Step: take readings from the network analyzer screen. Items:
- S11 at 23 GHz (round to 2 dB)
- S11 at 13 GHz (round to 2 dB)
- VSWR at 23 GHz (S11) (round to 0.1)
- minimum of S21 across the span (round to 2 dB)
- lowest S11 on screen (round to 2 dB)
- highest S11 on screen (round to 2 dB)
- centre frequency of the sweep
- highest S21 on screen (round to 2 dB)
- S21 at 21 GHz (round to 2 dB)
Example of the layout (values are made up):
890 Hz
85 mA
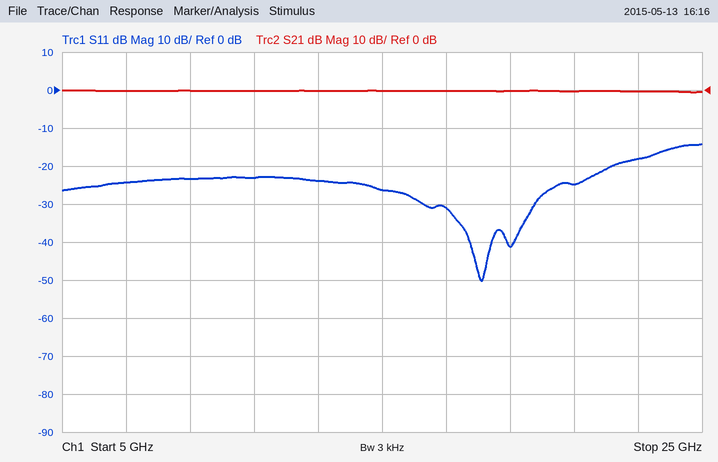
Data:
-18 dB
-24 dB
1.3
0 dB
-50 dB
-14 dB
15 GHz
0 dB
0 dB
